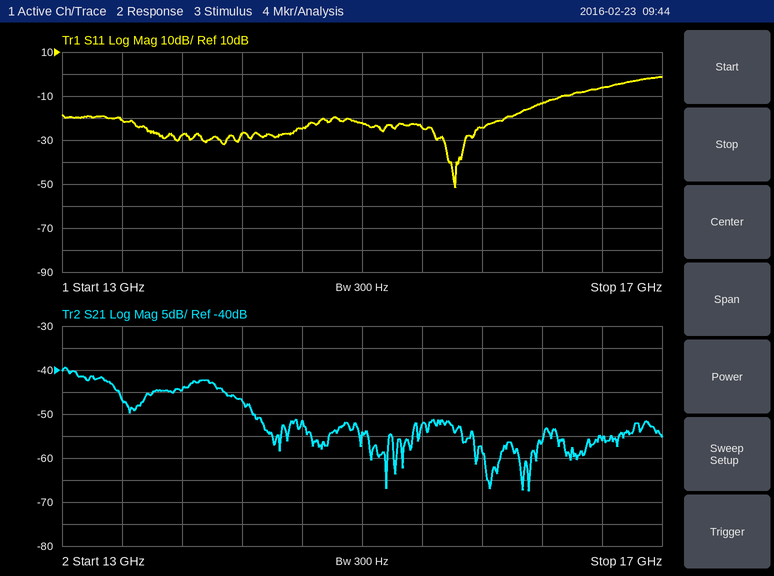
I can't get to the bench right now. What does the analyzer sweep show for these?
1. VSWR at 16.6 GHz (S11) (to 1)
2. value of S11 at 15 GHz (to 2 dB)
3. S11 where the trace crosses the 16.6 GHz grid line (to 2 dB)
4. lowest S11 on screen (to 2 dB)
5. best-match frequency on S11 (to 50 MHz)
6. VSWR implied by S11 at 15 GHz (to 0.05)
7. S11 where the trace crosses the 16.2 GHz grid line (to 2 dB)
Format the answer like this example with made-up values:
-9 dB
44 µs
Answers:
3
-22 dB
-6 dB
-52 dB
15.60 GHz
1.15
-14 dB
